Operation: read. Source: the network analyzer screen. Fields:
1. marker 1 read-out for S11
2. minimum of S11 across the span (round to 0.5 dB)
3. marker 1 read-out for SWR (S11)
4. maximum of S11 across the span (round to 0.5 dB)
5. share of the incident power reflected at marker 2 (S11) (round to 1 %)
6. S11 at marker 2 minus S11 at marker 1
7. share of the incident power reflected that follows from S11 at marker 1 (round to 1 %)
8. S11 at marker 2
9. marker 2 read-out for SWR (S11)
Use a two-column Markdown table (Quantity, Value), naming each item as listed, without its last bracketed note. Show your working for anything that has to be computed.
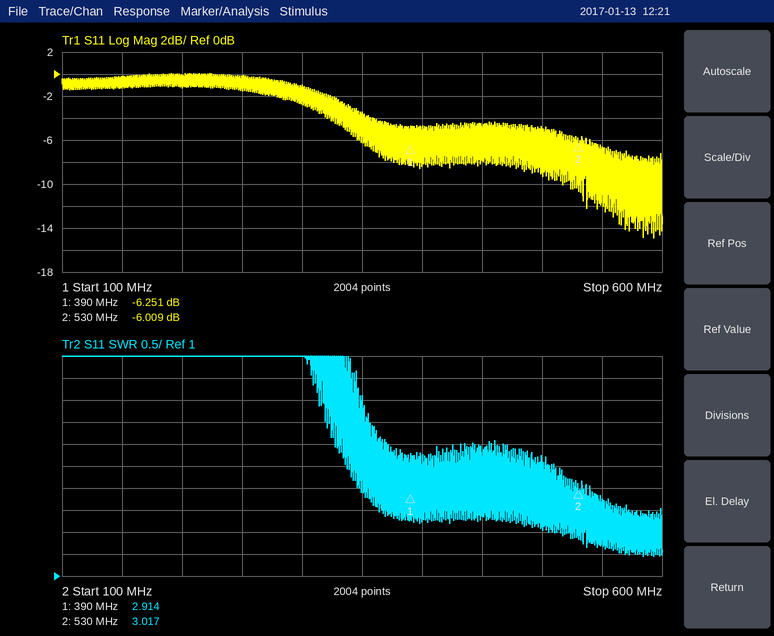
| Quantity | Value |
|---|---|
| marker 1 read-out for S11 | -6.251 dB |
| minimum of S11 across the span | -15.0 dB |
| marker 1 read-out for SWR | 2.914 |
| maximum of S11 across the span | 0.0 dB |
| share of the incident power reflected at marker 2 (S11) | 10^(-6.009/10) ≈ 25 % |
| S11 at marker 2 minus S11 at marker 1 | -6.009 − (-6.251) = 0.242 dB |
| share of the incident power reflected that follows from S11 at marker 1 | 10^(-6.251/10) ≈ 24 % |
| S11 at marker 2 | -6.009 dB |
| marker 2 read-out for SWR | 3.017 |
